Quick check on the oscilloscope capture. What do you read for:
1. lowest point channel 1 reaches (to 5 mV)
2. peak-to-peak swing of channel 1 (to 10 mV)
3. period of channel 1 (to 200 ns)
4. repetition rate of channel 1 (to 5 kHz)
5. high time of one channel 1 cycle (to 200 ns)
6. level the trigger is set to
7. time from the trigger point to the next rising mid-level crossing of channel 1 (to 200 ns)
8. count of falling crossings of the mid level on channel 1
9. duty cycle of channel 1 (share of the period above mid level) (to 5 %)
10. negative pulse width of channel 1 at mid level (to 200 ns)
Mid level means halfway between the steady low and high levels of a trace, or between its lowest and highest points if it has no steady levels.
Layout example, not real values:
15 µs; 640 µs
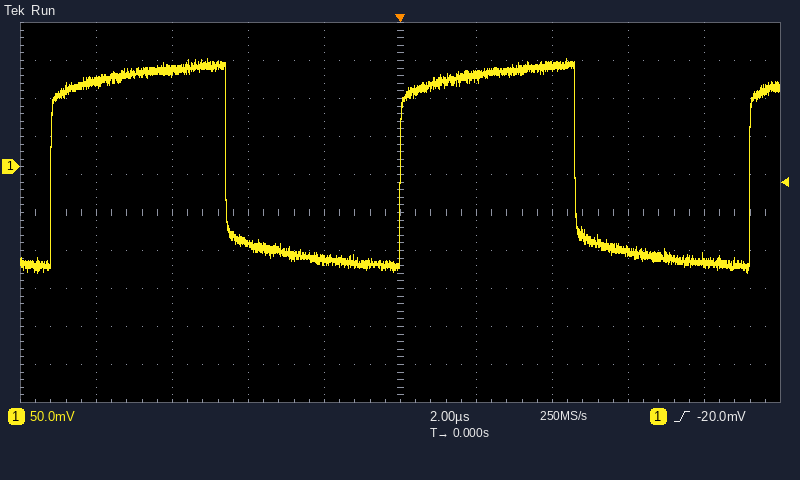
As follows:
-140 mV; 280 mV; 9.2 µs; 110 kHz; 4.6 µs; -20.0 mV; 9.2 µs; 2; 50 %; 4.6 µs
